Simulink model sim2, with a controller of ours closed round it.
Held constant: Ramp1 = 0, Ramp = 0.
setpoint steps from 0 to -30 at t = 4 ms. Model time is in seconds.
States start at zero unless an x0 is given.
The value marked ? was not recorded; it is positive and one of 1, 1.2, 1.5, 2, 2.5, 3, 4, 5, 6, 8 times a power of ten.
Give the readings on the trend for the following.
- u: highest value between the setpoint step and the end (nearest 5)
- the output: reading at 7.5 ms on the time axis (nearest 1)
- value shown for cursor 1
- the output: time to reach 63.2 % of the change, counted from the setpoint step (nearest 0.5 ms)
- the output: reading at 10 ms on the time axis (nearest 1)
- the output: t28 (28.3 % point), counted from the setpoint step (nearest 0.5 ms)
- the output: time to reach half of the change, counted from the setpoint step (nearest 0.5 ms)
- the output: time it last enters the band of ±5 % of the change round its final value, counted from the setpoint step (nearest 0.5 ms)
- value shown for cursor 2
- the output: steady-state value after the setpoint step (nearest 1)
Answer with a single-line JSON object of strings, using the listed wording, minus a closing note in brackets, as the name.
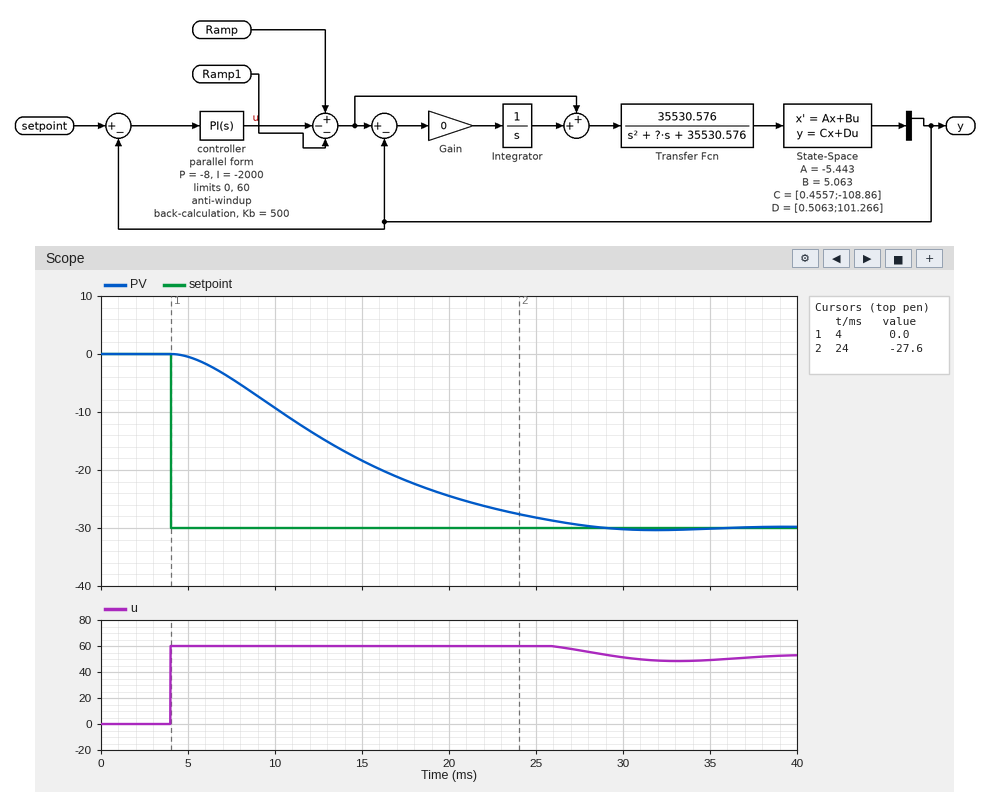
{"u: highest value between the setpoint step and the end": "60", "the output: reading at 7.5 ms on the time axis": "-4", "value shown for cursor 1": "0.0", "the output: time to reach 63.2 % of the change, counted from the setpoint step": "11.5 ms", "the output: reading at 10 ms on the time axis": "-9", "the output: t28 (28.3 % point), counted from the setpoint step": "5.5 ms", "the output: time to reach half of the change, counted from the setpoint step": "9.0 ms", "the output: time it last enters the band of ±5 % of the change round its final value, counted from the setpoint step": "21.5 ms", "value shown for cursor 2": "-27.6", "the output: steady-state value after the setpoint step": "-30"}
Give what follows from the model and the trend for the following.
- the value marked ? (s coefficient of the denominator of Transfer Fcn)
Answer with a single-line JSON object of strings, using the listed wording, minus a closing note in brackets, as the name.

{"the value marked ?": "400"}
